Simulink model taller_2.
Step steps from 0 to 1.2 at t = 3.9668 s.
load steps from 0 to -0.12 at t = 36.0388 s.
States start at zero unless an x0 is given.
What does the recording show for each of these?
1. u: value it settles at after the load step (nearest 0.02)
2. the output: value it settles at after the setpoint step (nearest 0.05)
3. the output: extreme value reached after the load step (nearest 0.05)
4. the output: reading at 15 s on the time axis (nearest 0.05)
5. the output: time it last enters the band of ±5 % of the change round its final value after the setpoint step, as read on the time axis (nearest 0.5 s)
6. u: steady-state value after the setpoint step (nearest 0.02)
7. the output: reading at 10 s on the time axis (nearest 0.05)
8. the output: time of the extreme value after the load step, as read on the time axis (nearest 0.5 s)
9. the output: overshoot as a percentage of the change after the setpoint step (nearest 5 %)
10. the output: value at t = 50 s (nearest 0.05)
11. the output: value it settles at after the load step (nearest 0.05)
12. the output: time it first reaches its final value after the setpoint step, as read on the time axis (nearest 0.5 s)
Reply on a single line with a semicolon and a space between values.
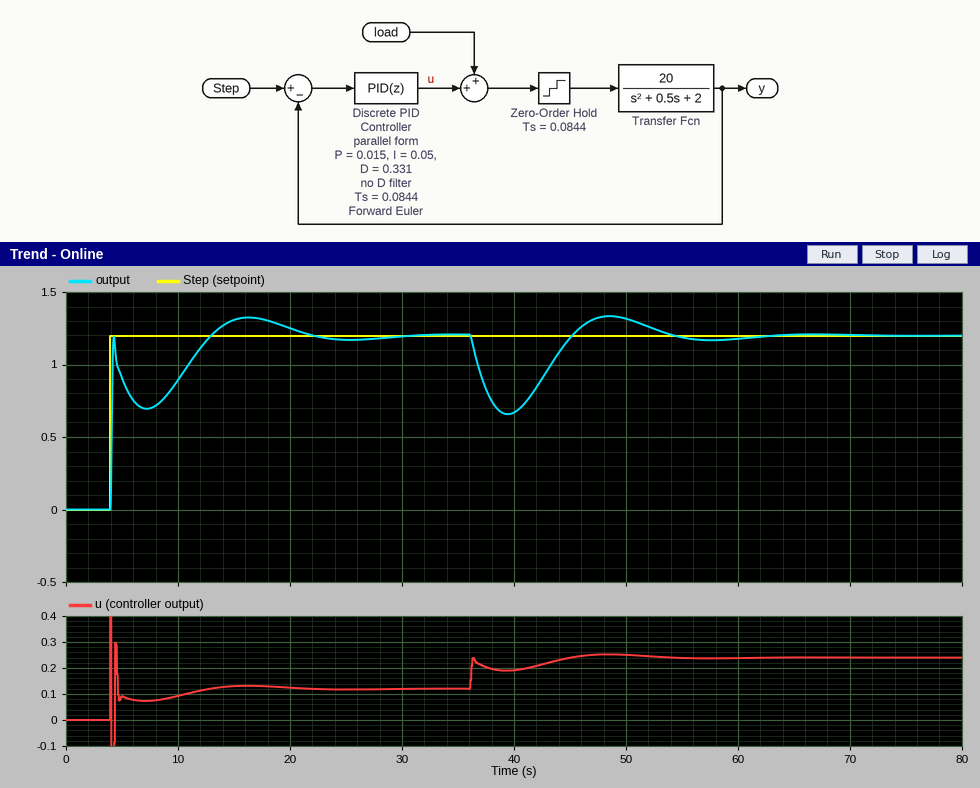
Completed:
0.24; 1.20; 0.65; 1.30; 19.5 s; 0.12; 0.90; 39.5 s; 10 %; 1.30; 1.20; 13.0 s
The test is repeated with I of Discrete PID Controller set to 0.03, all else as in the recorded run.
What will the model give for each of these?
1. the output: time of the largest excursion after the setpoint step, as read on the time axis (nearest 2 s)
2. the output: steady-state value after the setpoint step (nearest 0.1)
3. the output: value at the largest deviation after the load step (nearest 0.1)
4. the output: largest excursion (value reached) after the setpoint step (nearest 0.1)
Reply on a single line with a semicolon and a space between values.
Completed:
20 s; 1.2; 0.6; 1.3
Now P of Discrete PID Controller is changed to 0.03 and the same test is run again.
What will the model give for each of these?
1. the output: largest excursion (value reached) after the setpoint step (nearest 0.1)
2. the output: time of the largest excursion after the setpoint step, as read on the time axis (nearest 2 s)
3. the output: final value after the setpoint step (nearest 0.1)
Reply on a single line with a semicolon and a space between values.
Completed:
1.3; 16 s; 1.2
